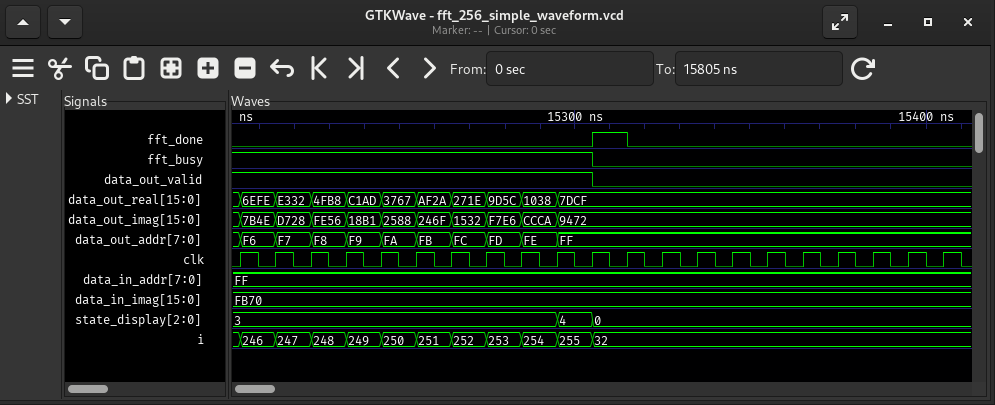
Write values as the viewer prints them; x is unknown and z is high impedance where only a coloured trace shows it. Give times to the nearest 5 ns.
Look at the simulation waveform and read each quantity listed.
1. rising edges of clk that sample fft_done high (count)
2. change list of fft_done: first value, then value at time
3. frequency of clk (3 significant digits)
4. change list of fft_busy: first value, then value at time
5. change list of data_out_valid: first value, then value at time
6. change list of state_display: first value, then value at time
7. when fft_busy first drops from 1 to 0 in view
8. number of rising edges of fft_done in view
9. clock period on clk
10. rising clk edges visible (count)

1
0, 1 at 15305 ns, 0 at 15315 ns
100 MHz
1, 0 at 15305 ns
1, 0 at 15305 ns
3, 4 at 15295 ns, 0 at 15305 ns
15305 ns
1
10 ns
21
